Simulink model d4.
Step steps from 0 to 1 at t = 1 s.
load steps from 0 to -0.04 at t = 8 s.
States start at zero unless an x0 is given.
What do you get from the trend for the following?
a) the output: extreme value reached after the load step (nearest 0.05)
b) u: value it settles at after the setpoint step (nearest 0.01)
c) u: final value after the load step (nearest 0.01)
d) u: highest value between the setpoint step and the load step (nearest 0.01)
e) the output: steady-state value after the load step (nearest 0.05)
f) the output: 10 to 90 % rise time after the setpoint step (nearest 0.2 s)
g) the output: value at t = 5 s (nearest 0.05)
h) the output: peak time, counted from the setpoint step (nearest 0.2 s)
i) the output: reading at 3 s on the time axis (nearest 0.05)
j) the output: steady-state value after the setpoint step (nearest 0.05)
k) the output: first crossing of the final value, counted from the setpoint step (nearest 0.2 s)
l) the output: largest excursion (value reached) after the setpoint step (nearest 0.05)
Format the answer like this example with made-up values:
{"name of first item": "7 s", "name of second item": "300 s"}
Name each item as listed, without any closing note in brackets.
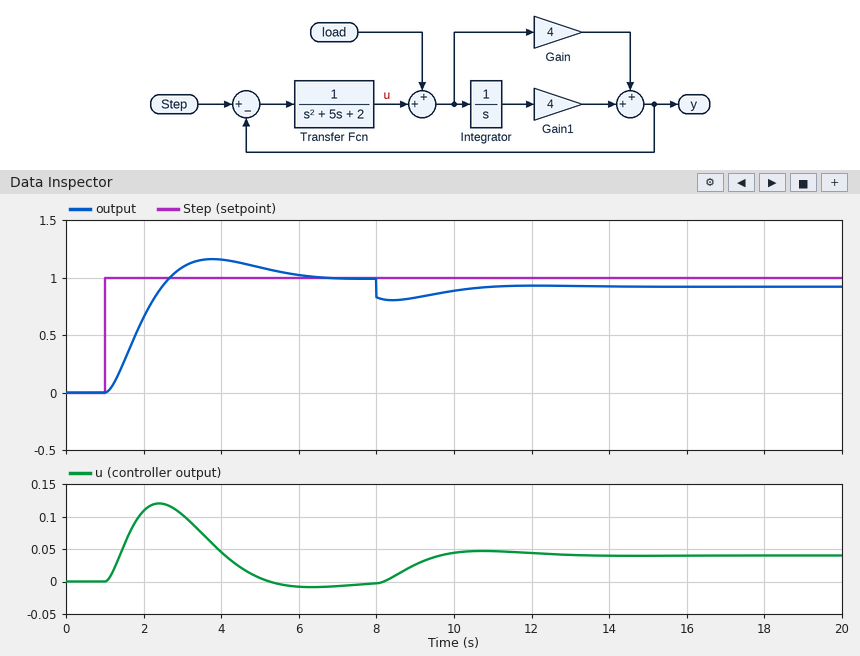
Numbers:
{"the output: extreme value reached after the load step": "0.80", "u: value it settles at after the setpoint step": "0.00", "u: final value after the load step": "0.04", "u: highest value between the setpoint step and the load step": "0.12", "the output: steady-state value after the load step": "0.90", "the output: 10 to 90 % rise time after the setpoint step": "1.2 s", "the output: value at t = 5 s": "1.10", "the output: peak time, counted from the setpoint step": "2.8 s", "the output: reading at 3 s on the time axis": "1.10", "the output: steady-state value after the setpoint step": "1.00", "the output: first crossing of the final value, counted from the setpoint step": "1.6 s", "the output: largest excursion (value reached) after the setpoint step": "1.15"}
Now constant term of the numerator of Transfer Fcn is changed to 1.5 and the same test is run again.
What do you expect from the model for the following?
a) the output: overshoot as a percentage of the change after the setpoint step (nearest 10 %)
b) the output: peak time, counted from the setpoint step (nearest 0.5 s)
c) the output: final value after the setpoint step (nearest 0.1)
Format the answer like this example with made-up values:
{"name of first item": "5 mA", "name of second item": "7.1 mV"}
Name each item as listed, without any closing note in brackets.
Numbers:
{"the output: overshoot as a percentage of the change after the setpoint step": "20 %", "the output: peak time, counted from the setpoint step": "2.0 s", "the output: final value after the setpoint step": "1.0"}
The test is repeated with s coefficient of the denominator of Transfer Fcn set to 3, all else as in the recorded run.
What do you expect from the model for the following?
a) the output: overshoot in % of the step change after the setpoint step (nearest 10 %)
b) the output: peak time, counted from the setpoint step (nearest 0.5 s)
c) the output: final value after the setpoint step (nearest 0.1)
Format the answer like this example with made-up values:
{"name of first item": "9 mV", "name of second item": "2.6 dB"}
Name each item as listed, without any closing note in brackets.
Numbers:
{"the output: overshoot in % of the step change after the setpoint step": "20 %", "the output: peak time, counted from the setpoint step": "2.0 s", "the output: final value after the setpoint step": "1.0"}
